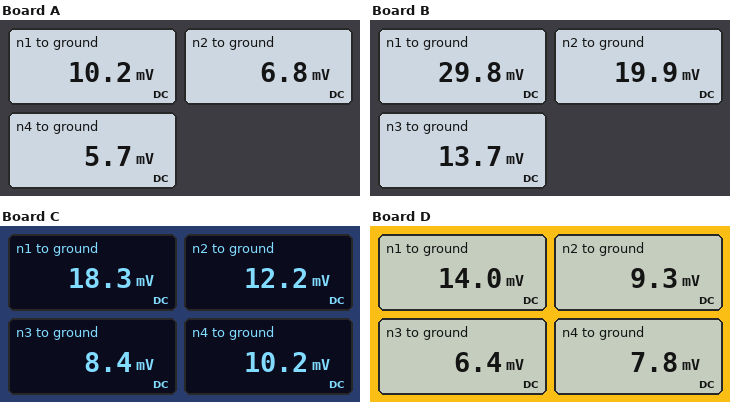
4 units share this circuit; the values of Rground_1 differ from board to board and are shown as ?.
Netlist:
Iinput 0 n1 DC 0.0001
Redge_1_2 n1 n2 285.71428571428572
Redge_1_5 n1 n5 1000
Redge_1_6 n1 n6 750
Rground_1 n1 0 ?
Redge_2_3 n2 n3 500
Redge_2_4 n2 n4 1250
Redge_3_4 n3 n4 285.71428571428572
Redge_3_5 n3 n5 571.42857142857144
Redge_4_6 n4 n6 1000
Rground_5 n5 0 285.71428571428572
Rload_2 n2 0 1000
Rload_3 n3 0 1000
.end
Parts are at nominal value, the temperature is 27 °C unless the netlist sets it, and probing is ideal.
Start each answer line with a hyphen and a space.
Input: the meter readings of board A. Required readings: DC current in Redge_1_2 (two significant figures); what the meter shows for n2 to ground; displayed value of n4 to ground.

- 12 µA
- 6.8 mV
- 5.7 mV
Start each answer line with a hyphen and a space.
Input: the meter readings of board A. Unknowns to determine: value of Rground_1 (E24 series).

- 130 Ω
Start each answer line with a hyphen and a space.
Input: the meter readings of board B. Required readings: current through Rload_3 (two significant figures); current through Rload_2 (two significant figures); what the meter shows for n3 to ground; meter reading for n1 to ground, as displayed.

- 14 µA
- 20 µA
- 13.7 mV
- 29.8 mV
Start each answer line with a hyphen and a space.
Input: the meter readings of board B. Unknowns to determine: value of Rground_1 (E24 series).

- 820 Ω
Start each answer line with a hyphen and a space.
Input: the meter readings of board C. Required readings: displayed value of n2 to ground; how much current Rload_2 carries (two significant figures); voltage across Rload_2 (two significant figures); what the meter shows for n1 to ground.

- 12.2 mV
- 12 µA
- 12 mV
- 18.3 mV
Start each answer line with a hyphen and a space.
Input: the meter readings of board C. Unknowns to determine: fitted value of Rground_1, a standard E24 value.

- 300 Ω
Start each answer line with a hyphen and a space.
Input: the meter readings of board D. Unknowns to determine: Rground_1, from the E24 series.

- 200 Ω
